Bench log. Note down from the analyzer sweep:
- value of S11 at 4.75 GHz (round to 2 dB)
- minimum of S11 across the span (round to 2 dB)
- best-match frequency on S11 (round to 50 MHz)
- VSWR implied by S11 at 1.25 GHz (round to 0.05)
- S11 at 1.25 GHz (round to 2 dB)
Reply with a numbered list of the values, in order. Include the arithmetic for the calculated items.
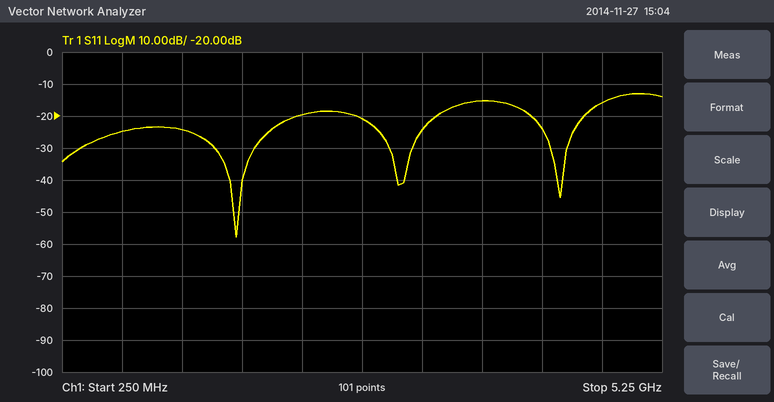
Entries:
1. -16 dB
2. -58 dB
3. 1.70 GHz
4. |Γ| = 10^(-24/20) = 0.0631; VSWR = (1 + 0.0631)/(1 − 0.0631) ≈ 1.13, so 1.15 to the nearest 0.05
5. -24 dB
